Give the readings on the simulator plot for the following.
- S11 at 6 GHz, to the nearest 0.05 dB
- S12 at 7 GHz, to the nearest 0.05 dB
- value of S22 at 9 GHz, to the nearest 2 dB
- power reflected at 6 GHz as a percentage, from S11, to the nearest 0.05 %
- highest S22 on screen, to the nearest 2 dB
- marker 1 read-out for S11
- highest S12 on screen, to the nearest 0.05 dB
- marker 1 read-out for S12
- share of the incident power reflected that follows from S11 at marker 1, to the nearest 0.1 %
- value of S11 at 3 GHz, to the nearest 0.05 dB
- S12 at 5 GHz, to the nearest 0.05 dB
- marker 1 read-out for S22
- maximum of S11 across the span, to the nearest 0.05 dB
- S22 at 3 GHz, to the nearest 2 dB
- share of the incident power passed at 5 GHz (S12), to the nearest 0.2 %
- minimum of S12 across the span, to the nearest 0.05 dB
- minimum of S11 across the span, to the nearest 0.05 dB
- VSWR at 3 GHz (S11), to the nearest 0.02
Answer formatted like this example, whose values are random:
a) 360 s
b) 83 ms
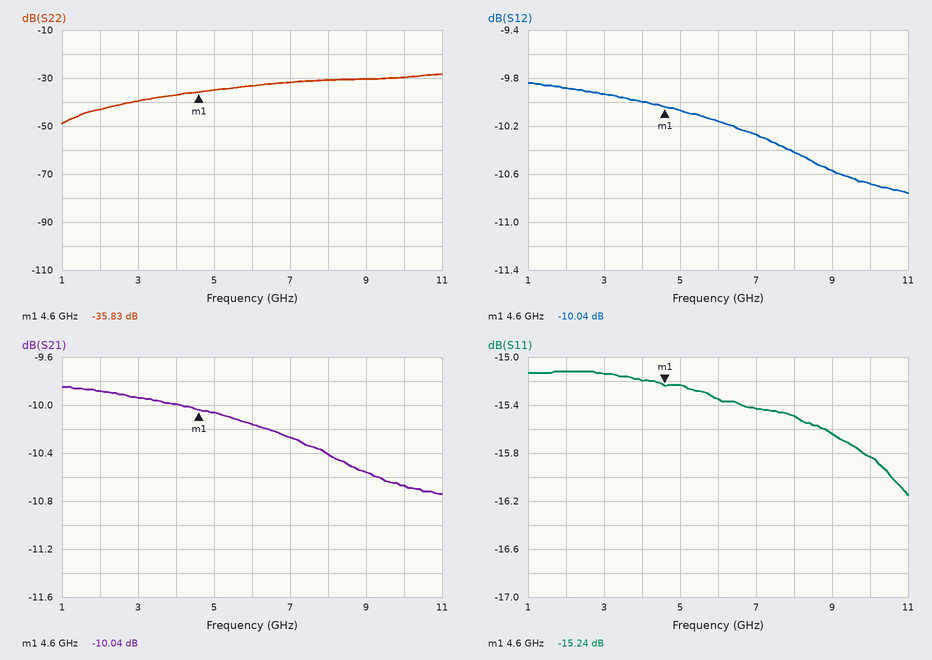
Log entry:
a) -15.35 dB
b) -10.25 dB
c) -30 dB
d) 2.90 %
e) -28 dB
f) -15.24 dB
g) -9.85 dB
h) -10.04 dB
i) 3.0 %
j) -15.15 dB
k) -10.05 dB
l) -35.83 dB
m) -15.10 dB
n) -40 dB
o) 9.8 %
p) -10.75 dB
q) -16.15 dB
r) 1.42
